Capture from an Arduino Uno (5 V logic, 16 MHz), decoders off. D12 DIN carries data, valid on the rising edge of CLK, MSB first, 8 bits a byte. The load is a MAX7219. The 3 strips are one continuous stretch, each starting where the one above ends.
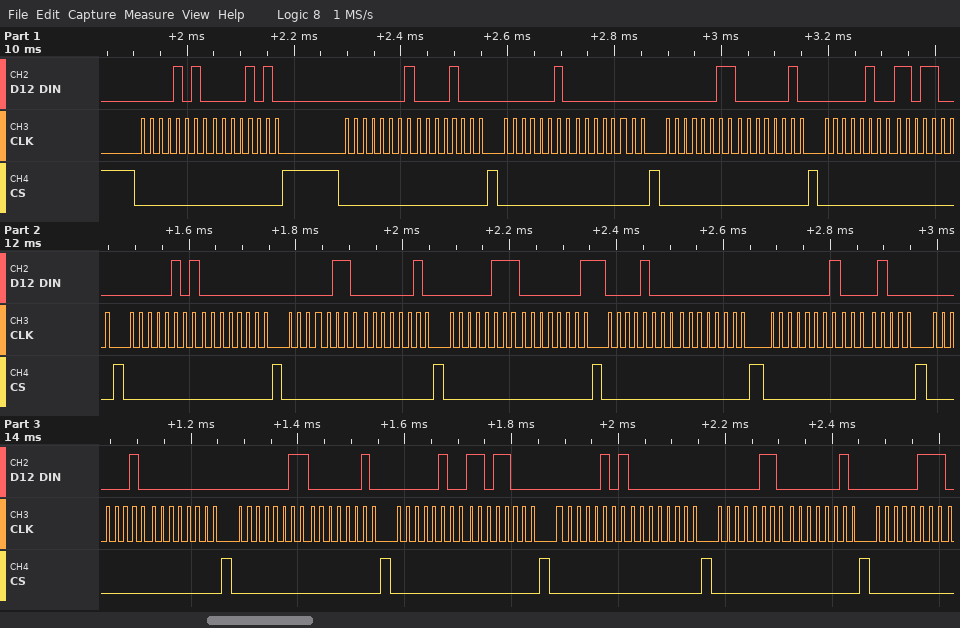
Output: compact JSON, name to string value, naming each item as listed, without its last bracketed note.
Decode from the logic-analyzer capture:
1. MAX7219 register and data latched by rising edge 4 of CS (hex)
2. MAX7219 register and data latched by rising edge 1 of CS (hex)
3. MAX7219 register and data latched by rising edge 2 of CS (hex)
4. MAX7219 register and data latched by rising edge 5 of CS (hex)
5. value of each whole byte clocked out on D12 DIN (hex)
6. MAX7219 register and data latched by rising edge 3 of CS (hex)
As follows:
{"MAX7219 register and data latched by rising edge 4 of CS": "register 0x3, data 0x02", "MAX7219 register and data latched by rising edge 1 of CS": "register 0xA, data 0x0A", "MAX7219 register and data latched by rising edge 2 of CS": "register 0x1, data 0x08", "MAX7219 register and data latched by rising edge 5 of CS": "register 0x4, data 0xD8", "value of each whole byte clocked out on D12 DIN": "0x0A 0x0A 0x01 0x08 0x02 0x00 0x03 0x02 0x04 0xD8 0x05 0x00 0x06 0x02 0x07 0x01 0x08 0x00 0x01 0x08 0x02 0x00 0x03 0x02 0x04 0xD8 0x05 0x00 0x06 0x02 0x07", "MAX7219 register and data latched by rising edge 3 of CS": "register 0x2, data 0x00"}
